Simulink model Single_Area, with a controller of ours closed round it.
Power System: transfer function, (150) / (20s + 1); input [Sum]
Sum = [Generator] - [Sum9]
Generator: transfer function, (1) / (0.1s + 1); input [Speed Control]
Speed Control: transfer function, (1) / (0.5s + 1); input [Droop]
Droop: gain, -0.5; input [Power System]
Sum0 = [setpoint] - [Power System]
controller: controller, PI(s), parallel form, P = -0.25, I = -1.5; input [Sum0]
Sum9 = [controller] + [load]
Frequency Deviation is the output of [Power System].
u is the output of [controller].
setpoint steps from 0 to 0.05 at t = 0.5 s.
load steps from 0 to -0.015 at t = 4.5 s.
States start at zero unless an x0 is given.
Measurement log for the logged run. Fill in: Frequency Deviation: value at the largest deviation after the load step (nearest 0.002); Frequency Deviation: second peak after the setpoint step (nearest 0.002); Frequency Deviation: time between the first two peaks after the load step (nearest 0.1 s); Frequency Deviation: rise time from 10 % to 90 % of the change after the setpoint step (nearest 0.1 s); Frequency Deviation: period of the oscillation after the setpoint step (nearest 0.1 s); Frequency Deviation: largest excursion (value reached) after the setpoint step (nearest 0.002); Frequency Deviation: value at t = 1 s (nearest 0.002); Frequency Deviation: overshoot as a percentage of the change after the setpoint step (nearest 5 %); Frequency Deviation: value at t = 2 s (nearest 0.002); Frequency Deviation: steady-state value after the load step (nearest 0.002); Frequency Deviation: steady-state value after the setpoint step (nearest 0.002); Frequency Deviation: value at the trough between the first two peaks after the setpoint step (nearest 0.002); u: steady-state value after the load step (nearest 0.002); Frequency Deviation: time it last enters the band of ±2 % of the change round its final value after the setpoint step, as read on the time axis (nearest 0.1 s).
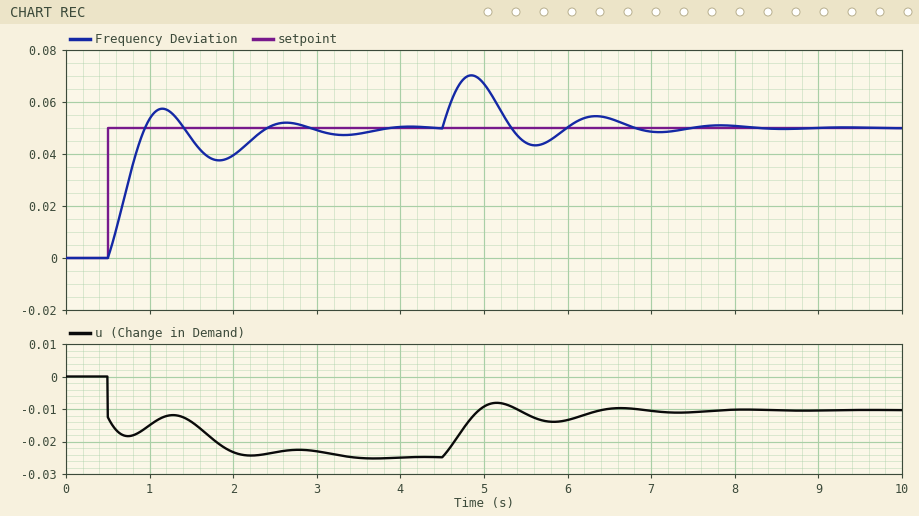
0.070
0.052
1.5 s
0.3 s
1.5 s
0.058
0.054
15 %
0.040
0.050
0.050
0.038
-0.010
3.7 s
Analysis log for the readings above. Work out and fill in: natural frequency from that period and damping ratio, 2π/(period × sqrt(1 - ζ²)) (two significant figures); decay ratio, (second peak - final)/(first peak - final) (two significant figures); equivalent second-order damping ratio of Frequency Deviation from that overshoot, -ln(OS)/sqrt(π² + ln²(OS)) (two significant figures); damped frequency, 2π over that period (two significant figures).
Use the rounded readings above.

4.9 rad/s
0.25
0.52
4.2 rad/s
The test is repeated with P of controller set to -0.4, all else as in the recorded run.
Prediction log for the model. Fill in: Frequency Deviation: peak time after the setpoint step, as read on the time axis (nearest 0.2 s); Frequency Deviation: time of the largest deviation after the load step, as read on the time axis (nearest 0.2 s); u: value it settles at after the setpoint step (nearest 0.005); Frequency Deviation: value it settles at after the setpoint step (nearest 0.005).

1.0 s
4.8 s
-0.025
0.050
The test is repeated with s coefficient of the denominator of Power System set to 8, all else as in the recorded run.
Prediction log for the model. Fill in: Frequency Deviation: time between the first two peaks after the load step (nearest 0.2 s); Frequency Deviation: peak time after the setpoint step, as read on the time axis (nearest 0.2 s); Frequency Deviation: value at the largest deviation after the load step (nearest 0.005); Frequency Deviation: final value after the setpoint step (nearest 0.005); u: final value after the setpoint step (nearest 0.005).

1.0 s
0.8 s
0.080
0.050
-0.025
